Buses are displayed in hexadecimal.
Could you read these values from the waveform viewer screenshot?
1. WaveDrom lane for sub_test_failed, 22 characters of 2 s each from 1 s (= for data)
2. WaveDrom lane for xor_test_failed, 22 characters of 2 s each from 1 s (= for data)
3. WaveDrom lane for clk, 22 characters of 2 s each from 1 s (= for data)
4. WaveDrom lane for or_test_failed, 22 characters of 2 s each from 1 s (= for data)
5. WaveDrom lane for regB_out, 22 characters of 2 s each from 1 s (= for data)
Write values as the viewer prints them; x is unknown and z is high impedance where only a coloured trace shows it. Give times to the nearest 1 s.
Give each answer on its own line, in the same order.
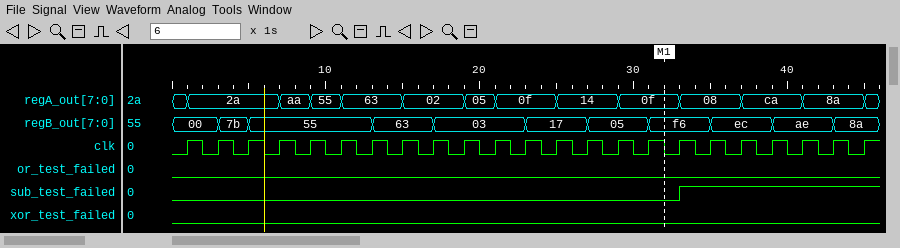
{name: 'sub_test_failed', wave: '0...............1.....'}
{name: 'xor_test_failed', wave: '0.....................'}
{name: 'clk', wave: 'p.....................'}
{name: 'or_test_failed', wave: '0.....................'}
{name: 'regB_out', wave: '===...=.=..=.=.=.=.=.=', data: '00 7b 55 63 03 17 05 f6 ec ae 8a'}
